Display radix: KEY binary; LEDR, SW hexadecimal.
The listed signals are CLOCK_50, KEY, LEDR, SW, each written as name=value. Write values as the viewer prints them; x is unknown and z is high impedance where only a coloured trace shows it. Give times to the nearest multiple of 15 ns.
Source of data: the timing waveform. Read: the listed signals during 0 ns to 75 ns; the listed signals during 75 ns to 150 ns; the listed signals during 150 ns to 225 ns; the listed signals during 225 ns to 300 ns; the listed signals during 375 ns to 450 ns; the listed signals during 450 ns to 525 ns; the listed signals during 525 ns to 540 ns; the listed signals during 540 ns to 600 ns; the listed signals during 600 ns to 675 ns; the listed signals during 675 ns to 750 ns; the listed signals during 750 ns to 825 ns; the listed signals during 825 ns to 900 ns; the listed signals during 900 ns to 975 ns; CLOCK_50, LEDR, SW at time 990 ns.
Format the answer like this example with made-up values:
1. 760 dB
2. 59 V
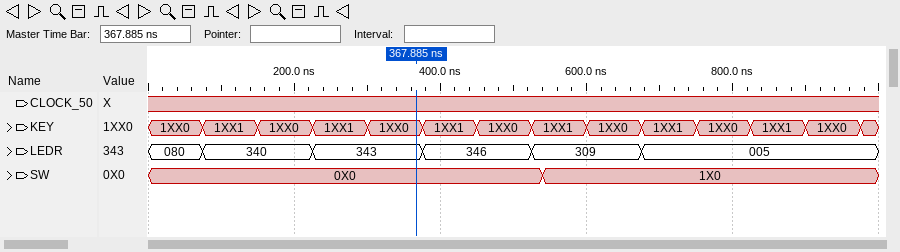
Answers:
1. CLOCK_50=x, KEY=1XX0, LEDR=080, SW=0X0
2. CLOCK_50=x, KEY=1XX1, LEDR=340, SW=0X0
3. CLOCK_50=x, KEY=1XX0, LEDR=340, SW=0X0
4. CLOCK_50=x, KEY=1XX1, LEDR=343, SW=0X0
5. CLOCK_50=x, KEY=1XX1, LEDR=346, SW=0X0
6. CLOCK_50=x, KEY=1XX0, LEDR=346, SW=0X0
7. CLOCK_50=x, KEY=1XX1, LEDR=309, SW=0X0
8. CLOCK_50=x, KEY=1XX1, LEDR=309, SW=1X0
9. CLOCK_50=x, KEY=1XX0, LEDR=309, SW=1X0
10. CLOCK_50=x, KEY=1XX1, LEDR=005, SW=1X0
11. CLOCK_50=x, KEY=1XX0, LEDR=005, SW=1X0
12. CLOCK_50=x, KEY=1XX1, LEDR=005, SW=1X0
13. CLOCK_50=x, KEY=1XX0, LEDR=005, SW=1X0
14. CLOCK_50=x, LEDR=005, SW=1X0
